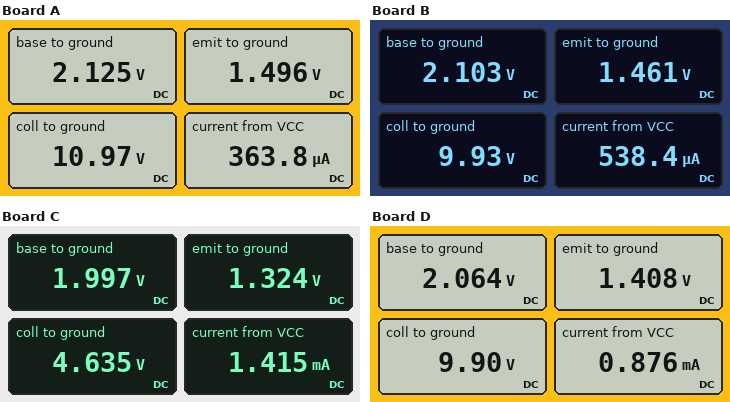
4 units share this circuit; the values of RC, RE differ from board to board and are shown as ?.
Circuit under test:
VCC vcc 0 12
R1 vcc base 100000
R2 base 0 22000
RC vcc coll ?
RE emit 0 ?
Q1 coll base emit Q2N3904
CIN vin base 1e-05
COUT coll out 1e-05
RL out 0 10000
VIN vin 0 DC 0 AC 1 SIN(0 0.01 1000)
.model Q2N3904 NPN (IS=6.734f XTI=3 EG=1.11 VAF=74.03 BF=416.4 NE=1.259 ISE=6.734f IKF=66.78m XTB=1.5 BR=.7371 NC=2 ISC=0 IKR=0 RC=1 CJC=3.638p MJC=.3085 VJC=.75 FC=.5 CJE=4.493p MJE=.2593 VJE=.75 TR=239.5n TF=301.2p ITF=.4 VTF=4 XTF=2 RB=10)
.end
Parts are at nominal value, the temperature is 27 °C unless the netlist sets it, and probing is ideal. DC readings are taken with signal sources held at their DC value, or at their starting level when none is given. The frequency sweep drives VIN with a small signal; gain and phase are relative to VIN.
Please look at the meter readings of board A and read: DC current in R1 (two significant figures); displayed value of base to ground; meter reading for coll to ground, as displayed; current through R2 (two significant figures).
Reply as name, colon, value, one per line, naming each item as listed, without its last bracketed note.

DC current in R1: 99 µA
displayed value of base to ground: 2.125 V
meter reading for coll to ground, as displayed: 10.97 V
current through R2: 97 µA
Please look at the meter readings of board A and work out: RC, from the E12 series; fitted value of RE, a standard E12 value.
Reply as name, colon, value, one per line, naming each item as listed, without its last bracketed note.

RC, from the E12 series: 3.9 kΩ
fitted value of RE, a standard E12 value: 5.6 kΩ
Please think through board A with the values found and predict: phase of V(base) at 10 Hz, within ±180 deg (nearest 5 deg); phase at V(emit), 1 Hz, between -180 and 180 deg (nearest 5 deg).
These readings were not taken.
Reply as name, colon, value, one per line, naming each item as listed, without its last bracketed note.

phase of V(base) at 10 Hz, within ±180 deg: 5 deg
phase at V(emit), 1 Hz, between -180 and 180 deg: 40 deg
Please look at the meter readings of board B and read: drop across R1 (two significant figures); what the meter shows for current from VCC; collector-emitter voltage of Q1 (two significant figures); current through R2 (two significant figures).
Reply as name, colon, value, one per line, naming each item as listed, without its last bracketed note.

drop across R1: 9.9 V
what the meter shows for current from VCC: 538.4 µA
collector-emitter voltage of Q1: 8.5 V
current through R2: 96 µA
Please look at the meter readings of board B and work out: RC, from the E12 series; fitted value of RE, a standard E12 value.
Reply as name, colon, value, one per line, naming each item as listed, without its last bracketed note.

RC, from the E12 series: 4.7 kΩ
fitted value of RE, a standard E12 value: 3.3 kΩ
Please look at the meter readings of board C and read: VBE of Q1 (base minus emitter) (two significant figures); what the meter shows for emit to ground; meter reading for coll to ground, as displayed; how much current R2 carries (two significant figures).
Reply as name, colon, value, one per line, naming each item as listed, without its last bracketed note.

VBE of Q1 (base minus emitter): 670 mV
what the meter shows for emit to ground: 1.324 V
meter reading for coll to ground, as displayed: 4.635 V
how much current R2 carries: 91 µA
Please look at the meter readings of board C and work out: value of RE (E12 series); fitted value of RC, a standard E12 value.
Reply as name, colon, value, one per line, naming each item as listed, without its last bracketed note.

value of RE: 1 kΩ
fitted value of RC, a standard E12 value: 5.6 kΩ
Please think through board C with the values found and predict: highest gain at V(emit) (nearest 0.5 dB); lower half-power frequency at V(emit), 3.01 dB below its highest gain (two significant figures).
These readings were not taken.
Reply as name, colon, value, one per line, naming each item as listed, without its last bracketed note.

highest gain at V(emit): 0 dB
lower half-power frequency at V(emit), 3.01 dB below its highest gain: 990 mHz
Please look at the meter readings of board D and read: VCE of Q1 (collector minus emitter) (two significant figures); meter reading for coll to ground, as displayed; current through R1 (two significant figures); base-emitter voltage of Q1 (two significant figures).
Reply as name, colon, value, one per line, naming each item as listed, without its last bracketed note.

VCE of Q1 (collector minus emitter): 8.5 V
meter reading for coll to ground, as displayed: 9.90 V
current through R1: 99 µA
base-emitter voltage of Q1: 660 mV
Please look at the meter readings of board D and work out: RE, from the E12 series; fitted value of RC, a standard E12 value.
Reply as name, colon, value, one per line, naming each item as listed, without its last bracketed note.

RE, from the E12 series: 1.8 kΩ
fitted value of RC, a standard E12 value: 2.7 kΩ
